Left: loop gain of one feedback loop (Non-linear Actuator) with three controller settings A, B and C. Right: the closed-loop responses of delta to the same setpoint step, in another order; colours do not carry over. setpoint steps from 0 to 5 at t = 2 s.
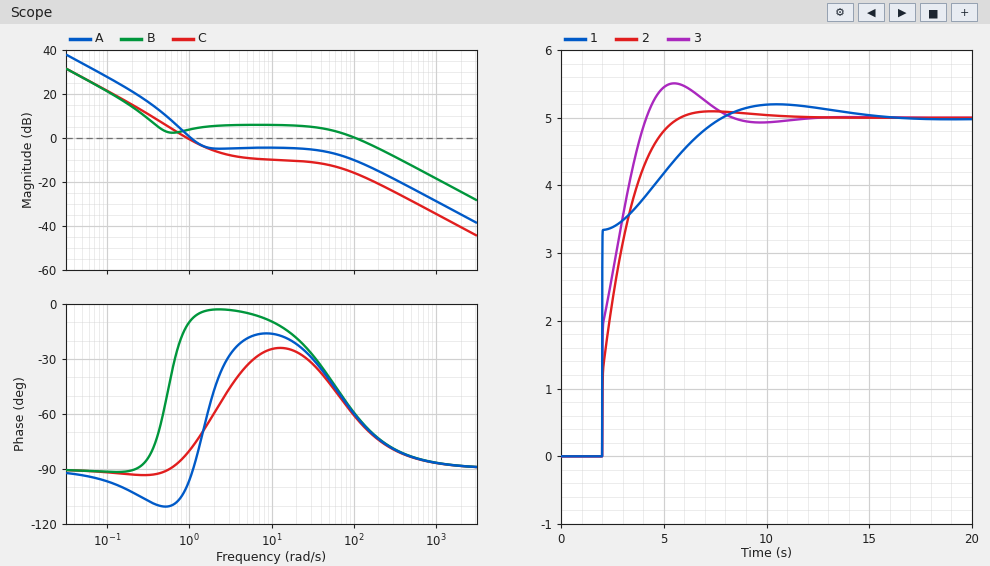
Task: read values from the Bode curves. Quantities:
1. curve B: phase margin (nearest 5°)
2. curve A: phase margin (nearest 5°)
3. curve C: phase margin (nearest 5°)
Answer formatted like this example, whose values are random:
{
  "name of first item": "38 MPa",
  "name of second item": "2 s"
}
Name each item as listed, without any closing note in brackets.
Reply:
{
  "curve B: phase margin": "120°",
  "curve A: phase margin": "85°",
  "curve C: phase margin": "100°"
}
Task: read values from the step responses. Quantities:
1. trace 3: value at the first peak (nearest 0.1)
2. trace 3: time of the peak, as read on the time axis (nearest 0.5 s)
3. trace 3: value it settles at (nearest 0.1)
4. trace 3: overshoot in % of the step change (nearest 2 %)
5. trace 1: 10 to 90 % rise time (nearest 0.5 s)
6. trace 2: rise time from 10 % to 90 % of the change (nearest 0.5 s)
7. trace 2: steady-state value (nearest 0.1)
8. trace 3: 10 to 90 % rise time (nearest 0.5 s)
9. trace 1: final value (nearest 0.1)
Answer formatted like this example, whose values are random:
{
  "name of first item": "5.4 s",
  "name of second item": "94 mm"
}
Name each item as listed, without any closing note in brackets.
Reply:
{
  "trace 3: value at the first peak": "5.5",
  "trace 3: time of the peak, as read on the time axis": "5.5 s",
  "trace 3: value it settles at": "5.0",
  "trace 3: overshoot in % of the step change": "10 %",
  "trace 1: 10 to 90 % rise time": "4.0 s",
  "trace 2: rise time from 10 % to 90 % of the change": "2.5 s",
  "trace 2: steady-state value": "5.0",
  "trace 3: 10 to 90 % rise time": "1.5 s",
  "trace 1: final value": "5.0"
}
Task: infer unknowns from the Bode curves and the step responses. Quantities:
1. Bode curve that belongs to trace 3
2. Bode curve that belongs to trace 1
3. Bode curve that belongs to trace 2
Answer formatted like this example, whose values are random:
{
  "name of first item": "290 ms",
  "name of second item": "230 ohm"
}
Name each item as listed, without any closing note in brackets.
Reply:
{
  "Bode curve that belongs to trace 3": "A",
  "Bode curve that belongs to trace 1": "B",
  "Bode curve that belongs to trace 2": "C"
}
